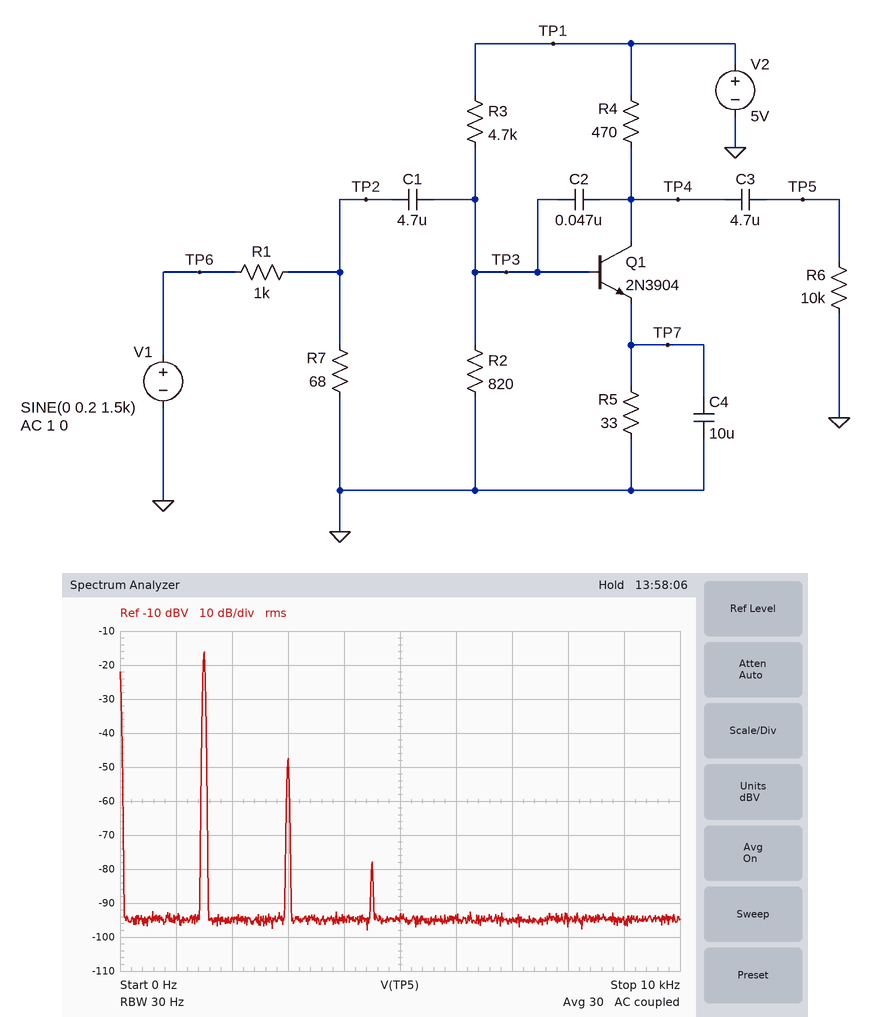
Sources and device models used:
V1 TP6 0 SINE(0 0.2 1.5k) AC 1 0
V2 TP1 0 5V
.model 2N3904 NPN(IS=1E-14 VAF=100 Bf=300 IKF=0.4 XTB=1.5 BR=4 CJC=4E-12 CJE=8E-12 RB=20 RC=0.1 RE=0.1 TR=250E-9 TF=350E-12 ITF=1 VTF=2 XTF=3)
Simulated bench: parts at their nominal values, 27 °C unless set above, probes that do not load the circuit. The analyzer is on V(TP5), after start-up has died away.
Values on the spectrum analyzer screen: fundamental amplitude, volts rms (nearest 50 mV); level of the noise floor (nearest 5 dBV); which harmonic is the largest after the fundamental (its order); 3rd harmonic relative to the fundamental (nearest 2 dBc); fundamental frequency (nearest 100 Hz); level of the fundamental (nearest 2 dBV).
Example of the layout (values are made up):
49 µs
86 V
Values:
150 mV
-95 dBV
2
-62 dBc
1.5 kHz
-16 dBV
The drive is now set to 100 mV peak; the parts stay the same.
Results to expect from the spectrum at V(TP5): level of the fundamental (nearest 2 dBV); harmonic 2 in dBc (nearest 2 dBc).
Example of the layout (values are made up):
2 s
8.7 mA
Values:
-22 dBV
-38 dBc
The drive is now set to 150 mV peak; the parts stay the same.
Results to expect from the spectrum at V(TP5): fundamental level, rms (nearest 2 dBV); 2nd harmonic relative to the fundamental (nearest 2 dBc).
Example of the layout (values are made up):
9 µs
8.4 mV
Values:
-18 dBV
-34 dBc
